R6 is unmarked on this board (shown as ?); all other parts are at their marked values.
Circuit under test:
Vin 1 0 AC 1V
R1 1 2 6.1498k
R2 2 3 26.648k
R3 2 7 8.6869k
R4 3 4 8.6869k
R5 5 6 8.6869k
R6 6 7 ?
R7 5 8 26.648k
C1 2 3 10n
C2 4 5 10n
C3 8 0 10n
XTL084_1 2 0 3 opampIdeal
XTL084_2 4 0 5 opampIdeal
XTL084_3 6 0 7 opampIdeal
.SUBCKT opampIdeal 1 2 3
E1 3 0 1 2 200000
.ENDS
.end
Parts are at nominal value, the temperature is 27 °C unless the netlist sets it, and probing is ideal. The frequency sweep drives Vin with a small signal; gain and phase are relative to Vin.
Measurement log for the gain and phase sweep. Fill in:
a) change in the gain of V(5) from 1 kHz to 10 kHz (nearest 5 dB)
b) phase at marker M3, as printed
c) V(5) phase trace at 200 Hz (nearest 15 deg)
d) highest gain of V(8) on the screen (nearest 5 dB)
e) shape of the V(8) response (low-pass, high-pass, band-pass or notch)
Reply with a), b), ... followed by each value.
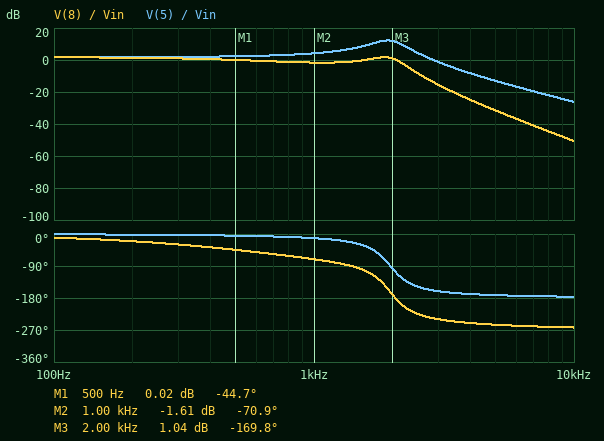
a) -30 dB
b) -169.8 deg
c) 0 deg
d) 0 dB
e) low-pass
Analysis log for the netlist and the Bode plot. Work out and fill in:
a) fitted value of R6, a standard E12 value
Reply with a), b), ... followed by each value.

a) 10 kΩ
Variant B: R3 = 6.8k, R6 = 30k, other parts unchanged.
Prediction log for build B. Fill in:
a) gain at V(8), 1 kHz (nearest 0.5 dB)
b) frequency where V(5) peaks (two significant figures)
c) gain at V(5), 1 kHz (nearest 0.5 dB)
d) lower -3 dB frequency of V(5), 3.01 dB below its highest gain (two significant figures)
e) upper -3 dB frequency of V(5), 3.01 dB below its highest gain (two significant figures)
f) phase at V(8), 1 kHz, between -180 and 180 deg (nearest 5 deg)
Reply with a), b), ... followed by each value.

a) -15.0 dB
b) 3.8 kHz
c) -9.5 dB
d) 3.5 kHz
e) 4.1 kHz
f) -60 deg
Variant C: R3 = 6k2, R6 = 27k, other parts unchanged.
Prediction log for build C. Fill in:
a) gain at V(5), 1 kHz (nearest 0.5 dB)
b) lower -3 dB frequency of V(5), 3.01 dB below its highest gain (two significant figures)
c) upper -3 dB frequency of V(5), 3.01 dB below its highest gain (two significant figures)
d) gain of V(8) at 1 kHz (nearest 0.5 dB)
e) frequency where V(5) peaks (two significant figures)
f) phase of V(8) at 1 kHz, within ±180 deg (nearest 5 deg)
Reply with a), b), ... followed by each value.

a) -9.0 dB
b) 3.5 kHz
c) 4.1 kHz
d) -15.0 dB
e) 3.8 kHz
f) -60 deg
